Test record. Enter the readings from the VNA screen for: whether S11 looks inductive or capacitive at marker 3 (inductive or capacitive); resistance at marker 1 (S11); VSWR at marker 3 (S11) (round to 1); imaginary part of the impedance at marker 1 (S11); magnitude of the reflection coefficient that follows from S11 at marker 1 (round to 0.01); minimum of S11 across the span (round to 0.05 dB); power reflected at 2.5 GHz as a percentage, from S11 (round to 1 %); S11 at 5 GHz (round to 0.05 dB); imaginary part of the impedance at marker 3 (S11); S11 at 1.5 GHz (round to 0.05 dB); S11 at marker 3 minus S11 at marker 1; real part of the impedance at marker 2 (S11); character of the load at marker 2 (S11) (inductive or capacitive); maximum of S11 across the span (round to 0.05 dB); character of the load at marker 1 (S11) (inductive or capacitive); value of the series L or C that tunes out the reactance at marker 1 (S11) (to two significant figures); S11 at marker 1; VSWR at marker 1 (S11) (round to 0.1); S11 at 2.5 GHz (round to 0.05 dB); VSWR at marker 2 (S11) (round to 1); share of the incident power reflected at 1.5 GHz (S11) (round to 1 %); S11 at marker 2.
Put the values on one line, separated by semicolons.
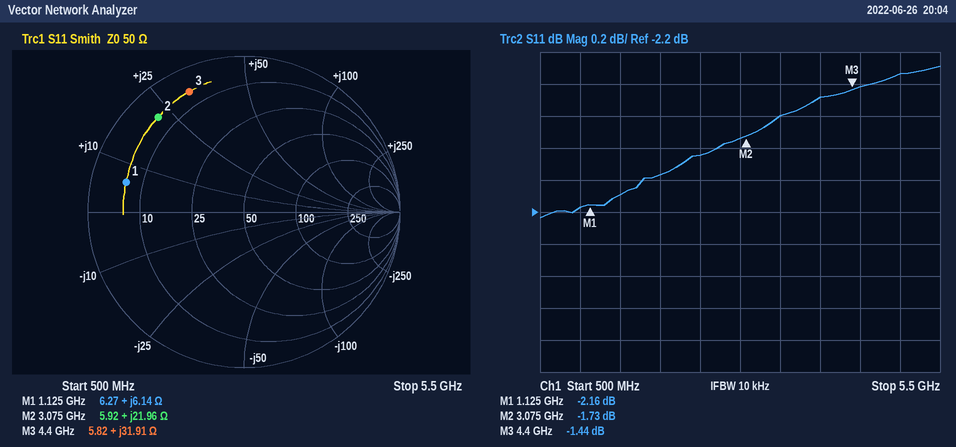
inductive; 6.27 Ω; 12; +6.14 Ω; 0.78; -2.25 dB; 65 %; -1.35 dB; +31.91 Ω; -2.10 dB; 0.72 dB; 5.92 Ω; inductive; -1.30 dB; inductive; 23 pF; -2.16 dB; 8.1; -1.85 dB; 10; 62 %; -1.73 dB
